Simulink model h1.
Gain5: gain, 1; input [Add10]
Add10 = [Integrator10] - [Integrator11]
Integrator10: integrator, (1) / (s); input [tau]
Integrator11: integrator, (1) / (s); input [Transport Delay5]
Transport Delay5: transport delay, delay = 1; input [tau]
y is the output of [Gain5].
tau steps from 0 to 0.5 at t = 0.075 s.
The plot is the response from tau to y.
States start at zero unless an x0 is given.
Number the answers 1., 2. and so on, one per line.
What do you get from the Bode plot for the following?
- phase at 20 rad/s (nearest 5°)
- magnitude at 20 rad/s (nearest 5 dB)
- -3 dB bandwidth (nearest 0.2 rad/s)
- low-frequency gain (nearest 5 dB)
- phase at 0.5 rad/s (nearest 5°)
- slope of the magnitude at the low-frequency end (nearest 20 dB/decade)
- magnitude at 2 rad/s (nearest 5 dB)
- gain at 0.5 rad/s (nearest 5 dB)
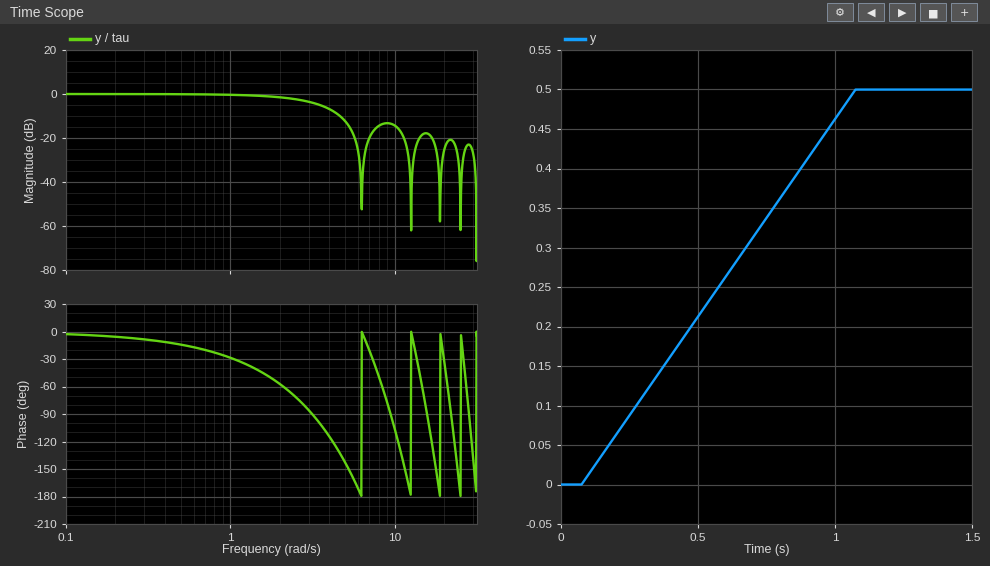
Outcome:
1. -35°
2. -25 dB
3. 2.8 rad/s
4. 0 dB
5. -15°
6. 0 dB/decade
7. 0 dB
8. 0 dB
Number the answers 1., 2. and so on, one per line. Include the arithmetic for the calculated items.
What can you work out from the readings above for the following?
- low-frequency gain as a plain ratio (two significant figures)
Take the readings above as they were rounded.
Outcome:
1. 10^(0 / 20) = 1.0
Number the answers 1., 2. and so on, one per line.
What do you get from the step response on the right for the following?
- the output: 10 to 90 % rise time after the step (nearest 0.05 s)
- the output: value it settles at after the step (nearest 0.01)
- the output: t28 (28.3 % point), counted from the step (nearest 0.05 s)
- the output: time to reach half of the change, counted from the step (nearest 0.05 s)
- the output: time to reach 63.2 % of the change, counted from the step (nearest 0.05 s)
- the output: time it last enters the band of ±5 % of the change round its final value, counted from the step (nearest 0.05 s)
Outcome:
1. 0.80 s
2. 0.50
3. 0.30 s
4. 0.50 s
5. 0.65 s
6. 0.95 s
